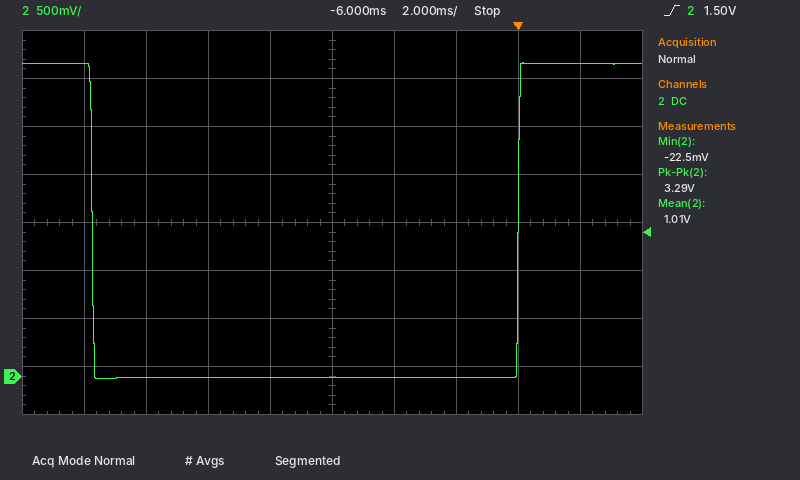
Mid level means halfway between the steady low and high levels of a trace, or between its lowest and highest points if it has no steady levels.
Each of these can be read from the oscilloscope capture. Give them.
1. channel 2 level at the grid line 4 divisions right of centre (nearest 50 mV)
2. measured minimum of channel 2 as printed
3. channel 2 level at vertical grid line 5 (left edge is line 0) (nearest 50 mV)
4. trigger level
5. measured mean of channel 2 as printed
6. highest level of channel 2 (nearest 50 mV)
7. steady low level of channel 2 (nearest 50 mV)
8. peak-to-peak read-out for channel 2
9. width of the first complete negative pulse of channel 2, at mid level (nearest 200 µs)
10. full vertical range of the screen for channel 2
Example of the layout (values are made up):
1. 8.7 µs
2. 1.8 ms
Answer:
1. 3.25 V
2. -22.5 mV
3. 0 mV
4. 1.50 V
5. 1.01 V
6. 3.25 V
7. 0 mV
8. 3.29 V
9. 13.8 ms
10. 4 V
